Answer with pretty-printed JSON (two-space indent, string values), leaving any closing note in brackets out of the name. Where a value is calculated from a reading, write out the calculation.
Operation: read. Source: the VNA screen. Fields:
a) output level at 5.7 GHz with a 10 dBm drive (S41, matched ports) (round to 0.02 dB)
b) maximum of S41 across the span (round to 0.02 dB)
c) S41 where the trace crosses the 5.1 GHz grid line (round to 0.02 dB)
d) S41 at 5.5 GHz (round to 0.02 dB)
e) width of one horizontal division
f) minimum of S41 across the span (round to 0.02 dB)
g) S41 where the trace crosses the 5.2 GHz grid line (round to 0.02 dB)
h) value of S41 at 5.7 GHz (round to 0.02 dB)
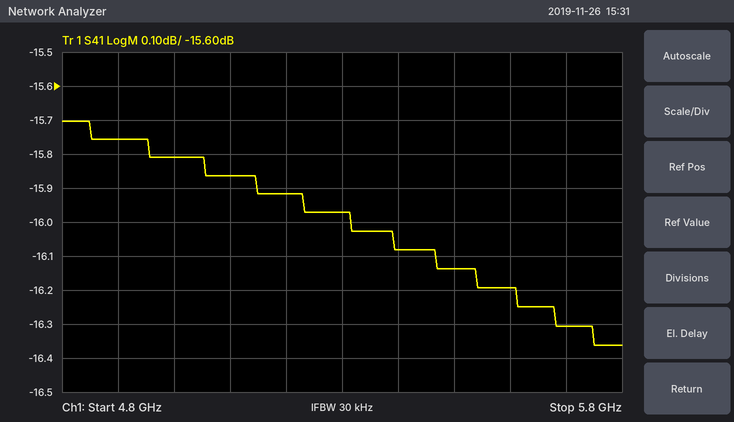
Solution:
{
  "output level at 5.7 GHz with a 10 dBm drive (S41, matched ports)": "10 dBm + (-16.30 dB) = -6.30 dBm",
  "maximum of S41 across the span": "-15.70 dB",
  "S41 where the trace crosses the 5.1 GHz grid line": "-15.86 dB",
  "S41 at 5.5 GHz": "-16.14 dB",
  "width of one horizontal division": "100 MHz",
  "minimum of S41 across the span": "-16.36 dB",
  "S41 where the trace crosses the 5.2 GHz grid line": "-15.92 dB",
  "value of S41 at 5.7 GHz": "-16.30 dB"
}
